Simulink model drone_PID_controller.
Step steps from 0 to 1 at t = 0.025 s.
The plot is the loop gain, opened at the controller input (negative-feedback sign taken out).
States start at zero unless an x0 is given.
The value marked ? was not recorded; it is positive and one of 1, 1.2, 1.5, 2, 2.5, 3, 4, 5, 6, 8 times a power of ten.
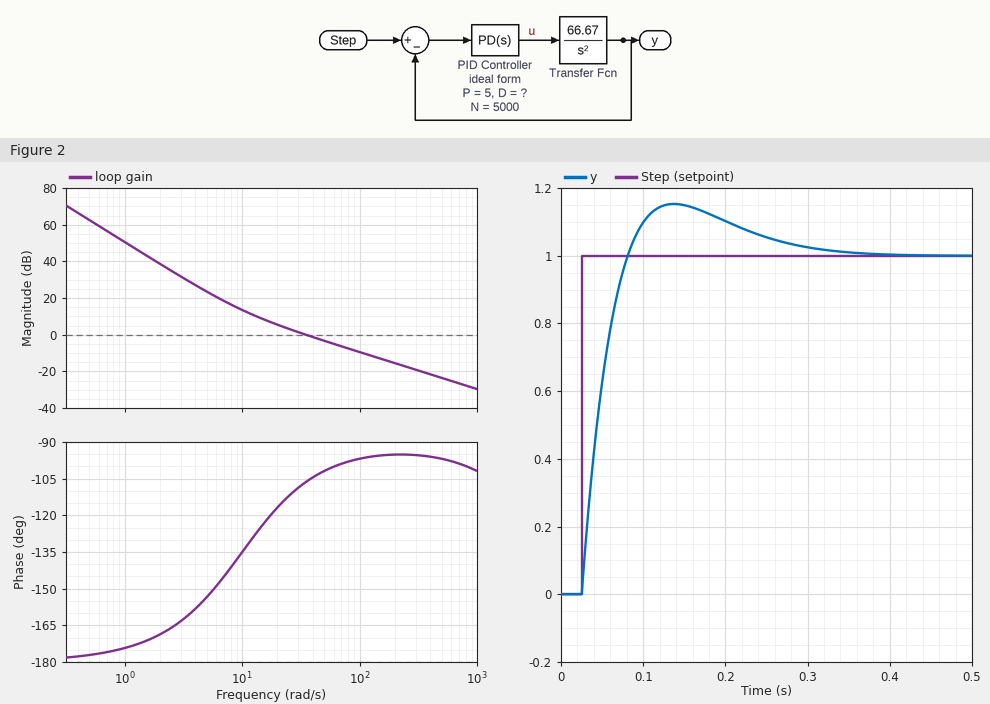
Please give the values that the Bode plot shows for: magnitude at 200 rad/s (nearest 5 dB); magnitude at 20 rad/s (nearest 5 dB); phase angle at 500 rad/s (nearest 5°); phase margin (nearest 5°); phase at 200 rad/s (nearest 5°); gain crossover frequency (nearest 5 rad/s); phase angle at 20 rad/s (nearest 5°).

-15 dB
5 dB
-95°
75°
-95°
35 rad/s
-115°
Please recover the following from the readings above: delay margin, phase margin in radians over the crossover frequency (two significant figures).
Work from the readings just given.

0.037 s
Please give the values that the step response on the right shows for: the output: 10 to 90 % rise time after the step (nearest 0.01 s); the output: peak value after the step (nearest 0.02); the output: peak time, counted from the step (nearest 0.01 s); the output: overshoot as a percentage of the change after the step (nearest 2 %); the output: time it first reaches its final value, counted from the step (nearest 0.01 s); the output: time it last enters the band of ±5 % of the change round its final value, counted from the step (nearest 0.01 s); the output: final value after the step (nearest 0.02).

0.04 s
1.16
0.11 s
16 %
0.06 s
0.23 s
1.00
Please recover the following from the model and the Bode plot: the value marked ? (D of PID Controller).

0.1
